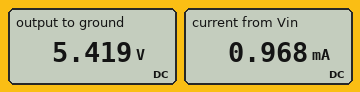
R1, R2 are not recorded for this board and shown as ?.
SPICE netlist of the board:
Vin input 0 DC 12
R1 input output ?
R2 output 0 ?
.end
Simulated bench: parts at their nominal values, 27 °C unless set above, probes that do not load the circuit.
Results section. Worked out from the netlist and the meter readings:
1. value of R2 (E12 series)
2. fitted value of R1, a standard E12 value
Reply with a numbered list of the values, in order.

1. 5.6 kΩ
2. 6.8 kΩ
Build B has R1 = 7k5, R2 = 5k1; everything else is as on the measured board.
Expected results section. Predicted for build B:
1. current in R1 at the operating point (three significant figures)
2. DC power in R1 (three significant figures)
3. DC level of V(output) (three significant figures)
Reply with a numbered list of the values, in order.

1. 952 µA
2. 6.80 mW
3. 4.86 V
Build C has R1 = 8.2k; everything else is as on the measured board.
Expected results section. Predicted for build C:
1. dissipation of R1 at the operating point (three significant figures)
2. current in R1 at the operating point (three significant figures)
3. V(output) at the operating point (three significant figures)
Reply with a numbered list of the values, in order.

1. 6.20 mW
2. 870 µA
3. 4.87 V
